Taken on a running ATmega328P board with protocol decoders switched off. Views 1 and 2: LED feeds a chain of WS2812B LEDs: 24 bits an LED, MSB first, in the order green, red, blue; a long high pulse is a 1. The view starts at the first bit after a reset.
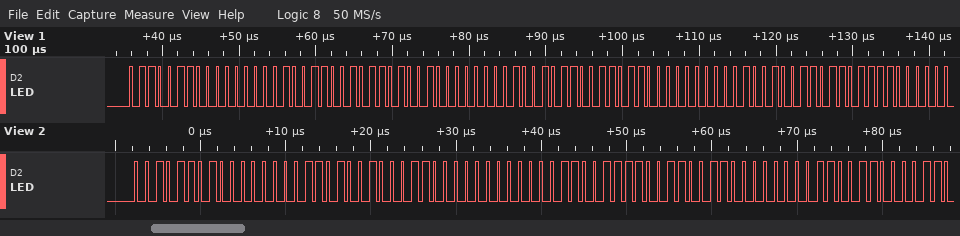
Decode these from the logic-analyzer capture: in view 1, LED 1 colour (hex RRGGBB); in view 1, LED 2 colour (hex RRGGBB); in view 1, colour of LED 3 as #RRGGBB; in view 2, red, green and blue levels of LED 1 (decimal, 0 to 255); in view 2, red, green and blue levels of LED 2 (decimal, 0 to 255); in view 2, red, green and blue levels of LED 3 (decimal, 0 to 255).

#006699
#006996
#006C93
0, 45, 210
0, 48, 207
0, 51, 204
